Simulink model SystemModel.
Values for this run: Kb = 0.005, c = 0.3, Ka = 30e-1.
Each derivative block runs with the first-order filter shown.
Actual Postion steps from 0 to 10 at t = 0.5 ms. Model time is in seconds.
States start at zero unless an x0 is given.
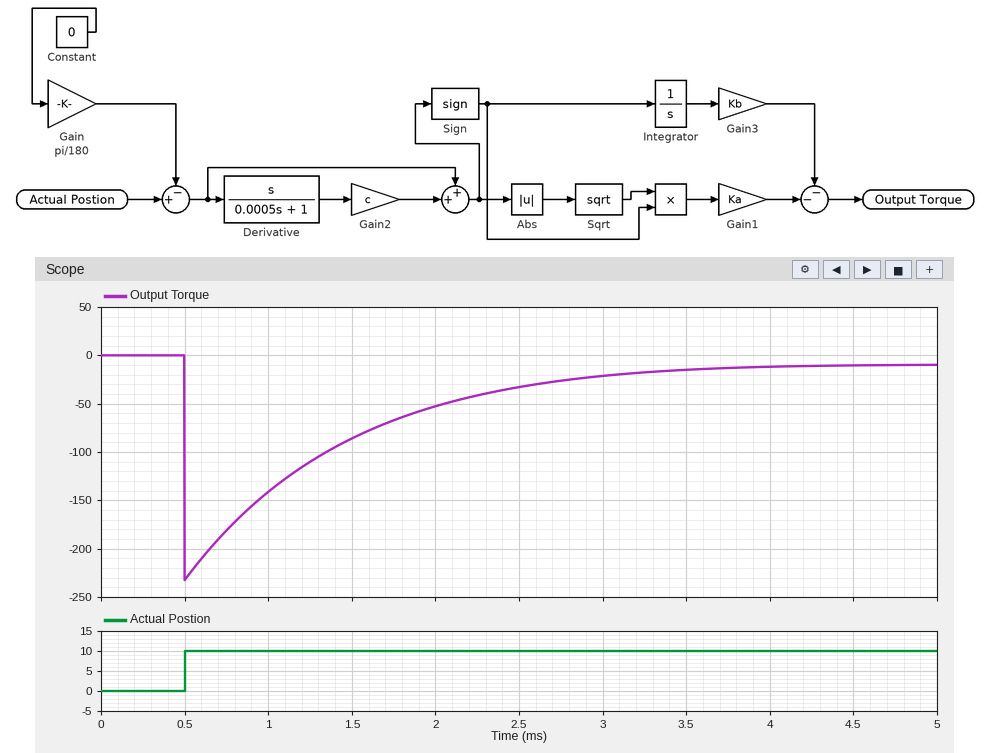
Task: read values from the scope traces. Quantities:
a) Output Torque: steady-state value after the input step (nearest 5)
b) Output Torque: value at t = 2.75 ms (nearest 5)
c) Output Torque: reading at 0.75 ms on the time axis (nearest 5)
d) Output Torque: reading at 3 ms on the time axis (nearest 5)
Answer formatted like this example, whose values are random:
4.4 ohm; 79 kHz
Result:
-10; -25; -180; -20
